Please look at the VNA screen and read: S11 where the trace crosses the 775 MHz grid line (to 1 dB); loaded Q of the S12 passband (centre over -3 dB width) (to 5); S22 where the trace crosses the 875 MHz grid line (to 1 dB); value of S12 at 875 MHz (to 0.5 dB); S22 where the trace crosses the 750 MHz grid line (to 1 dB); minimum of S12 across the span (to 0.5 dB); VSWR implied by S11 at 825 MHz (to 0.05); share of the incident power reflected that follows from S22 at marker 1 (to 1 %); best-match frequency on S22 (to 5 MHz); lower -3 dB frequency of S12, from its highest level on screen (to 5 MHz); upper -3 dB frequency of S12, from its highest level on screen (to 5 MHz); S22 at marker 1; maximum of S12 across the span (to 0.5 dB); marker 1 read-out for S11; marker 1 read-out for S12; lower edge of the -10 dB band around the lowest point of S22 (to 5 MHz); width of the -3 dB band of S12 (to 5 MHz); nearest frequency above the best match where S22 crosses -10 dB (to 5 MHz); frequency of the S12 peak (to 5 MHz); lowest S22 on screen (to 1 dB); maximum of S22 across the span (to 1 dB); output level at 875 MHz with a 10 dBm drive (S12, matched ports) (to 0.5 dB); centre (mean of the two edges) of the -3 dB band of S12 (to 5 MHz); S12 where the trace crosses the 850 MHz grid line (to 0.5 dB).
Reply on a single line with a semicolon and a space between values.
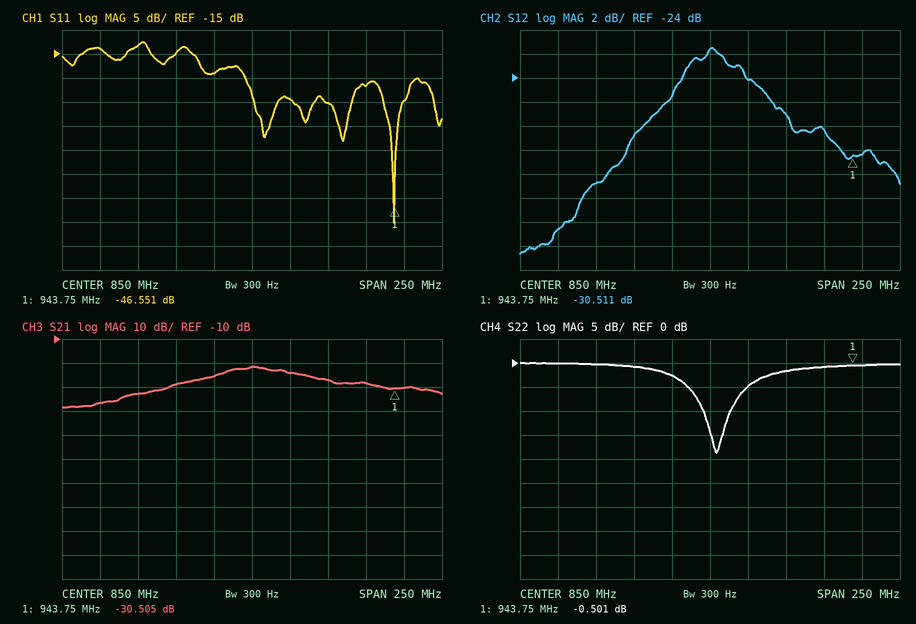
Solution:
-13 dB; 15; -5 dB; -24.0 dB; 0 dB; -38.5 dB; 1.25; 89 %; 855 MHz; 830 MHz; 880 MHz; -0.501 dB; -21.5 dB; -46.551 dB; -30.511 dB; 845 MHz; 50 MHz; 865 MHz; 850 MHz; -19 dB; 0 dB; -14.0 dBm; 855 MHz; -21.5 dB
